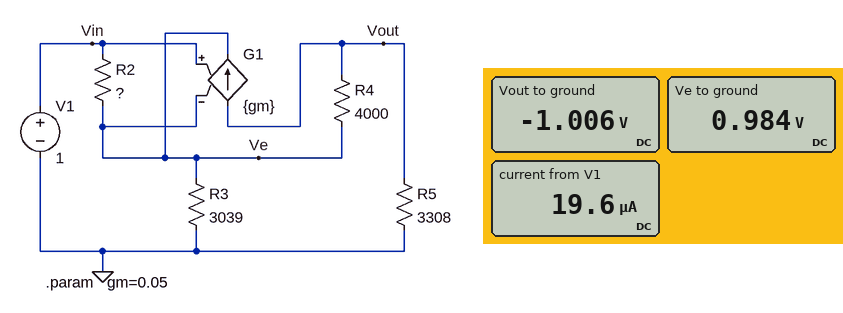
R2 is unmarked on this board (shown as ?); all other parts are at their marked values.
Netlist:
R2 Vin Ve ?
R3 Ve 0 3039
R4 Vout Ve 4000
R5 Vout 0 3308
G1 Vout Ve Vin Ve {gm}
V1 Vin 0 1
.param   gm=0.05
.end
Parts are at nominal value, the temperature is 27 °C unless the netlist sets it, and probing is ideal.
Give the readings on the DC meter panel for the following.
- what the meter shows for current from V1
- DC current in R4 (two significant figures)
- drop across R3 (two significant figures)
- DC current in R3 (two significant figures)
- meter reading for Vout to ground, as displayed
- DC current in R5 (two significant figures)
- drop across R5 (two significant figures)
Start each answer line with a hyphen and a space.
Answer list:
- 19.6 µA
- 500 µA
- 980 mV
- 320 µA
- -1.006 V
- 300 µA
- 1.0 V
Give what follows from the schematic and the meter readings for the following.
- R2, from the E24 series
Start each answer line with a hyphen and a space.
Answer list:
- 820 Ω
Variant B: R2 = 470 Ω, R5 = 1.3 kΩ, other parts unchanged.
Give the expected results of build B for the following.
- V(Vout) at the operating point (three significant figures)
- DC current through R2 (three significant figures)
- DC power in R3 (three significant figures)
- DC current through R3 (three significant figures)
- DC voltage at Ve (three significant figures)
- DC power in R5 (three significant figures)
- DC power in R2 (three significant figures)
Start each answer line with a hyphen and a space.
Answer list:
- -387 mV
- 27.3 µA
- 321 µW
- 325 µA
- 987 mV
- 115 µW
- 350 nW
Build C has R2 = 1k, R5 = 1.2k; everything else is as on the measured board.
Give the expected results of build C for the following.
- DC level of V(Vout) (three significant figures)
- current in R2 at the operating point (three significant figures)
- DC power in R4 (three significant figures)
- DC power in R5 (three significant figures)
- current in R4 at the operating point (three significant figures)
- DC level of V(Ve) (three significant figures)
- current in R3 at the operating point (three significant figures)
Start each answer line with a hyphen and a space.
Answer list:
- -374 mV
- 13.0 µA
- 463 µW
- 117 µW
- 340 µA
- 987 mV
- 325 µA
